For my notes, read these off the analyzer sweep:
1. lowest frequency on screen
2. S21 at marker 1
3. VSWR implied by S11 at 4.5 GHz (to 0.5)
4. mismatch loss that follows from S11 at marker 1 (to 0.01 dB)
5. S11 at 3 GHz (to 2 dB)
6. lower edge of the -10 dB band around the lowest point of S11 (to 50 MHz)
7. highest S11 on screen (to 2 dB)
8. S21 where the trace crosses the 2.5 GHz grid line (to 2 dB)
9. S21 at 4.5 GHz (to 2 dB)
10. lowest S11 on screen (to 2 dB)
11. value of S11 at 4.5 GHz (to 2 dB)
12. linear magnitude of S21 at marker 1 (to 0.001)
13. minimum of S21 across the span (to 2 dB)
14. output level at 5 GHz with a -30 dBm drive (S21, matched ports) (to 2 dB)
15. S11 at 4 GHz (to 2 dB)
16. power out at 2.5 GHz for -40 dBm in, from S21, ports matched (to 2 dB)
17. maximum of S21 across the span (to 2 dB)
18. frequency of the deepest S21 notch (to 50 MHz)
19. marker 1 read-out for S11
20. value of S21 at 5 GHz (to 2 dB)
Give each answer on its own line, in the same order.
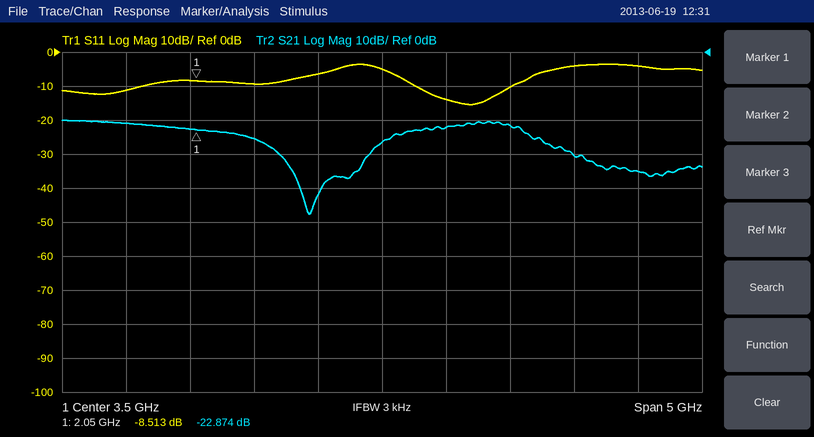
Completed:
1 GHz
-22.874 dB
2.0
0.66 dB
-6 dB
3.75 GHz
-4 dB
-26 dB
-22 dB
-16 dB
-10 dB
0.072
-48 dB
-60 dBm
-14 dB
-66 dBm
-20 dB
2.95 GHz
-8.513 dB
-30 dB
